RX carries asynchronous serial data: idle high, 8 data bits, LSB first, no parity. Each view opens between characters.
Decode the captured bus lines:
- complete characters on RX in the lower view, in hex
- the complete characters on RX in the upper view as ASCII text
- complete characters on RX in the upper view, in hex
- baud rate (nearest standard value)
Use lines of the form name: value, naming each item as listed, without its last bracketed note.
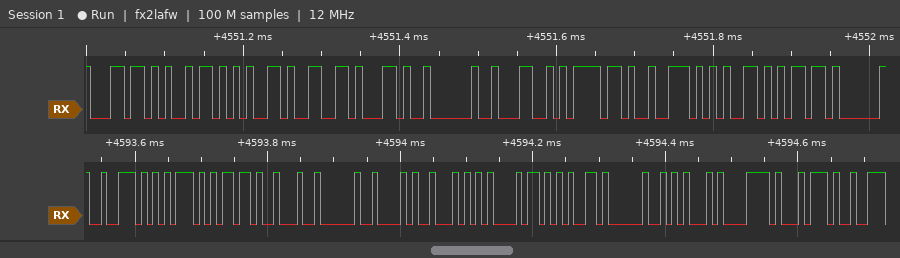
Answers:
complete characters on RX in the lower view, in hex: 72, 75, 6D, 22, 20, 28, 54, 68, 65, 20, 45, 78, 74
the complete characters on RX in the upper view as ASCII text: "lief, Lorem"
complete characters on RX in the upper view, in hex: 6C, 69, 65, 66, 2C, 20, 4C, 6F, 72, 65, 6D
baud rate: 115200 baud
